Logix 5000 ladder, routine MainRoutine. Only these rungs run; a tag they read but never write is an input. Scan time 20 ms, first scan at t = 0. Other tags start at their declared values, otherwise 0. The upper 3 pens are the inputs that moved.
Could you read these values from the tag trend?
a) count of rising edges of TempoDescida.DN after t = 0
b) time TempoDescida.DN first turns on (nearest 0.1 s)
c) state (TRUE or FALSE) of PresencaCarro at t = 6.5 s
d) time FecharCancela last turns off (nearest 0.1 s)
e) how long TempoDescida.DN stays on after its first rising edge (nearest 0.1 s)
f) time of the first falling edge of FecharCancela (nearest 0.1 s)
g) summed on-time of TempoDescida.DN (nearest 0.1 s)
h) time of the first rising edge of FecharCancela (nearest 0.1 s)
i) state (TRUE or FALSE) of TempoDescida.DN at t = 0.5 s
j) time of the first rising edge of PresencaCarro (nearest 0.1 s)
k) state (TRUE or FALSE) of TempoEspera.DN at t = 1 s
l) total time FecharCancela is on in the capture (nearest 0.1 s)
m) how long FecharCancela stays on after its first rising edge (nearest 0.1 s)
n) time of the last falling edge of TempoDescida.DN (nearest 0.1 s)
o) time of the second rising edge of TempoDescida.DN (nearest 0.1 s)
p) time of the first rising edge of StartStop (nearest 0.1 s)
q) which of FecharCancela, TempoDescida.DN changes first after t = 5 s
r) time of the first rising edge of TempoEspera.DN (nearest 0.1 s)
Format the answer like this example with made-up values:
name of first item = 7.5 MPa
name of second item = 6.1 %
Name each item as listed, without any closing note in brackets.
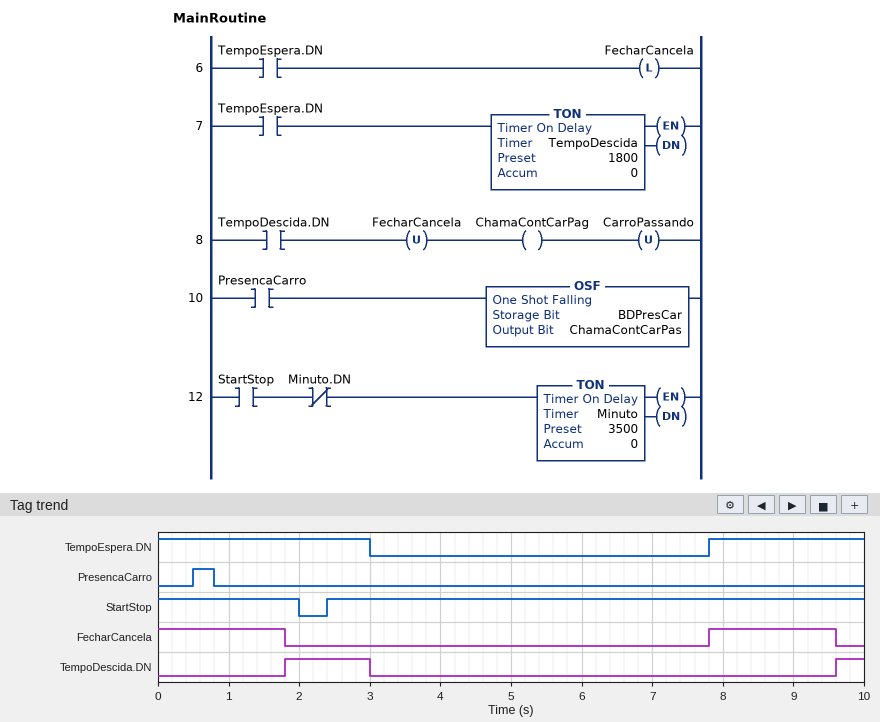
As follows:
count of rising edges of TempoDescida.DN after t = 0 = 2
time TempoDescida.DN first turns on = 1.8 s
state (TRUE or FALSE) of PresencaCarro at t = 6.5 s = FALSE
time FecharCancela last turns off = 9.6 s
how long TempoDescida.DN stays on after its first rising edge = 1.2 s
time of the first falling edge of FecharCancela = 1.8 s
summed on-time of TempoDescida.DN = 1.6 s
time of the first rising edge of FecharCancela = 7.8 s
state (TRUE or FALSE) of TempoDescida.DN at t = 0.5 s = FALSE
time of the first rising edge of PresencaCarro = 0.5 s
state (TRUE or FALSE) of TempoEspera.DN at t = 1 s = TRUE
total time FecharCancela is on in the capture = 3.6 s
how long FecharCancela stays on after its first rising edge = 1.8 s
time of the last falling edge of TempoDescida.DN = 3.0 s
time of the second rising edge of TempoDescida.DN = 9.6 s
time of the first rising edge of StartStop = 2.4 s
which of FecharCancela, TempoDescida.DN changes first after t = 5 s = FecharCancela
time of the first rising edge of TempoEspera.DN = 7.8 s
